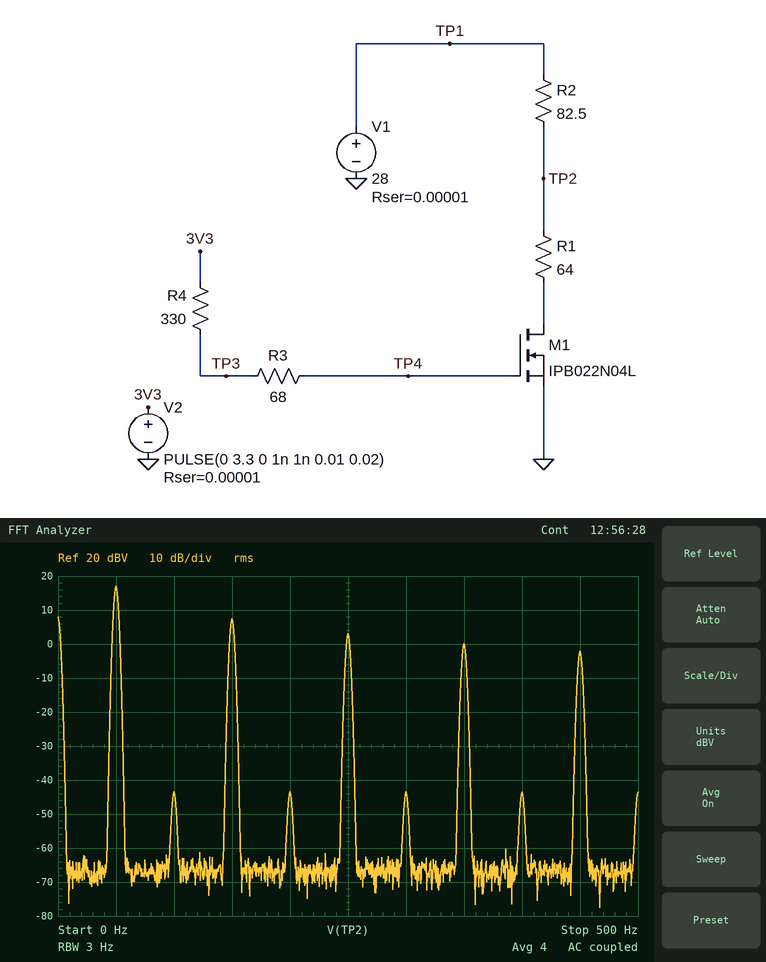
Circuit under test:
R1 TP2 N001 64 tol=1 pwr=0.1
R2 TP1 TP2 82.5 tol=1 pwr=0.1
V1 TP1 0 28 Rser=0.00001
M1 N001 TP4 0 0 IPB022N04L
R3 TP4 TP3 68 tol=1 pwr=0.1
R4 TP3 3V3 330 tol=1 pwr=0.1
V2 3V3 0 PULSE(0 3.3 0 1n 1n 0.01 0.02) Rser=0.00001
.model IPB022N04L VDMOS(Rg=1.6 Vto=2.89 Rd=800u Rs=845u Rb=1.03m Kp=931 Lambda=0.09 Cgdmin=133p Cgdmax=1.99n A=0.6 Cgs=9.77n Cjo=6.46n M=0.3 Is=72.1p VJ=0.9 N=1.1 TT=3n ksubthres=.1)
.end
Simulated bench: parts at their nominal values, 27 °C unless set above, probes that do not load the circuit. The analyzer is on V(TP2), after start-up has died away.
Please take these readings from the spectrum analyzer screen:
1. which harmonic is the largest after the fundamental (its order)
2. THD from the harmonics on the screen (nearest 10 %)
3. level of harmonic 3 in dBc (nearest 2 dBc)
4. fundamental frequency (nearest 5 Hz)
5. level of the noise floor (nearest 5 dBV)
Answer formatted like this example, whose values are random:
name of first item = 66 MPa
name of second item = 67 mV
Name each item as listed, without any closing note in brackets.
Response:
which harmonic is the largest after the fundamental = 3
THD from the harmonics on the screen = 40 %
level of harmonic 3 in dBc = -10 dBc
fundamental frequency = 50 Hz
level of the noise floor = -65 dBV
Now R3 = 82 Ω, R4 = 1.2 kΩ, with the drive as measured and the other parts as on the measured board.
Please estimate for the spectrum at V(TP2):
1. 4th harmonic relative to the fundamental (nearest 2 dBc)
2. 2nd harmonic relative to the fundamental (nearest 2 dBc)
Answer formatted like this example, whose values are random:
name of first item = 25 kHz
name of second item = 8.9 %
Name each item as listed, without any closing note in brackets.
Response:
4th harmonic relative to the fundamental = -50 dBc
2nd harmonic relative to the fundamental = -50 dBc
